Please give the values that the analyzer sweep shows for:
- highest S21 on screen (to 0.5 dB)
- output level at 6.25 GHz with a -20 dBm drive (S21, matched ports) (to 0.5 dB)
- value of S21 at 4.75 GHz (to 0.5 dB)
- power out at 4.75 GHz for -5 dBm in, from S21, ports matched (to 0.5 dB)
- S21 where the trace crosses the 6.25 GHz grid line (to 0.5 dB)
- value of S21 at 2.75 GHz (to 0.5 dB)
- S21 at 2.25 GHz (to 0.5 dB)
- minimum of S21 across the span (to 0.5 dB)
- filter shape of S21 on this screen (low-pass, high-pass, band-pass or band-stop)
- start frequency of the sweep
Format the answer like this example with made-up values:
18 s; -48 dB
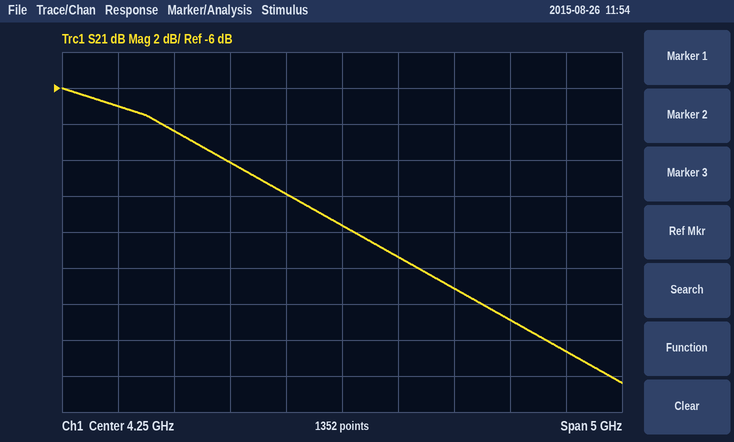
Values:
-6.0 dB; -40.5 dBm; -15.5 dB; -20.5 dBm; -20.5 dB; -8.5 dB; -7.0 dB; -22.5 dB; low-pass; 1.75 GHz
